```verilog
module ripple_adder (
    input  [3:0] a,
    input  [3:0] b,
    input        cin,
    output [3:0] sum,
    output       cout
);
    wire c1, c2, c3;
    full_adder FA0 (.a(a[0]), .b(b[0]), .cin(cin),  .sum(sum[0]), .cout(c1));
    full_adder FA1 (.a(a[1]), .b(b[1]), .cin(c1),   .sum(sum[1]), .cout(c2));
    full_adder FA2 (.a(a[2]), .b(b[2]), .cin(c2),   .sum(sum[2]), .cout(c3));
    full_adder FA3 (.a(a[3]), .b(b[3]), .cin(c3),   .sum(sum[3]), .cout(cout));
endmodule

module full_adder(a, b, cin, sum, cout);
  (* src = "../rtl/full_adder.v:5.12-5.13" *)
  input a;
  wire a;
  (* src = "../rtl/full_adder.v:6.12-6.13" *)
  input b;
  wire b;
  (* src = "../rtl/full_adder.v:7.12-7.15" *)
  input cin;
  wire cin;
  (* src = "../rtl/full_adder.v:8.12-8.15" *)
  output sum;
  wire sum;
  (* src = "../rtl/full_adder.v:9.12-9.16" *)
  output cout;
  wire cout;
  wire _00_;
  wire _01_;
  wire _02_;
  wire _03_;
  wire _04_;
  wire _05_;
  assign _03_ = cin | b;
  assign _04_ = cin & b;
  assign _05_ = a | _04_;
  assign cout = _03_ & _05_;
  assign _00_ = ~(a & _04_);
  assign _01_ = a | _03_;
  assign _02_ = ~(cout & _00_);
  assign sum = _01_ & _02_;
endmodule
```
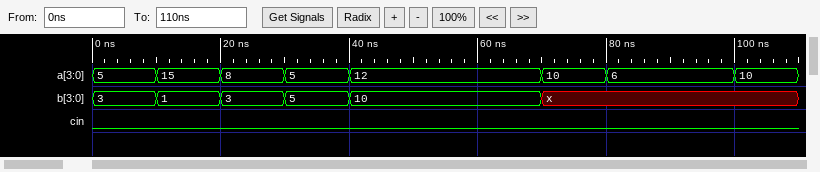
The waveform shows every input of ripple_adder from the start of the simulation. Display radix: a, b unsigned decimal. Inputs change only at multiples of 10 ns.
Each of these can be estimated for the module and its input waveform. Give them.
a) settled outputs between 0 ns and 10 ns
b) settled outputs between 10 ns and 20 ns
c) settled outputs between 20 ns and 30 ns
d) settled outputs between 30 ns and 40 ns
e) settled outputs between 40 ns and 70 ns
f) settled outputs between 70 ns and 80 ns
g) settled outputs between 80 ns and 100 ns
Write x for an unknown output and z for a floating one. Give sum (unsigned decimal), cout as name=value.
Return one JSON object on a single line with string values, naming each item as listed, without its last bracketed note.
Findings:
{"settled outputs between 0 ns and 10 ns": "sum=8, cout=0", "settled outputs between 10 ns and 20 ns": "sum=0, cout=1", "settled outputs between 20 ns and 30 ns": "sum=11, cout=0", "settled outputs between 30 ns and 40 ns": "sum=10, cout=0", "settled outputs between 40 ns and 70 ns": "sum=6, cout=1", "settled outputs between 70 ns and 80 ns": "sum=x, cout=x", "settled outputs between 80 ns and 100 ns": "sum=x, cout=x"}
